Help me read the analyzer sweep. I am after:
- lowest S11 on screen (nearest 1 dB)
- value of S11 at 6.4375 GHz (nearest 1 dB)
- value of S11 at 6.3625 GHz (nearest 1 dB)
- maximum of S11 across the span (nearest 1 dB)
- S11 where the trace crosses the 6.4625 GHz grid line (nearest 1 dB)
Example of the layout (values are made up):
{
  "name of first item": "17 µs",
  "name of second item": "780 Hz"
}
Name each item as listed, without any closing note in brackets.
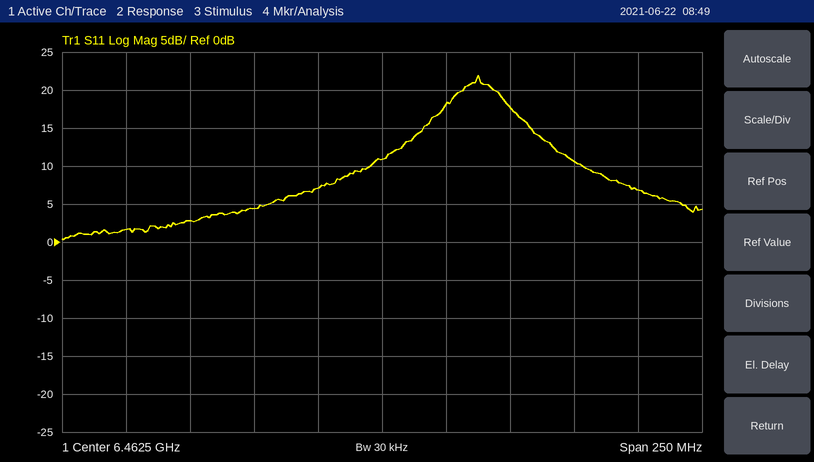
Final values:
{
  "lowest S11 on screen": "0 dB",
  "value of S11 at 6.4375 GHz": "7 dB",
  "value of S11 at 6.3625 GHz": "2 dB",
  "maximum of S11 across the span": "22 dB",
  "S11 where the trace crosses the 6.4625 GHz grid line": "11 dB"
}
